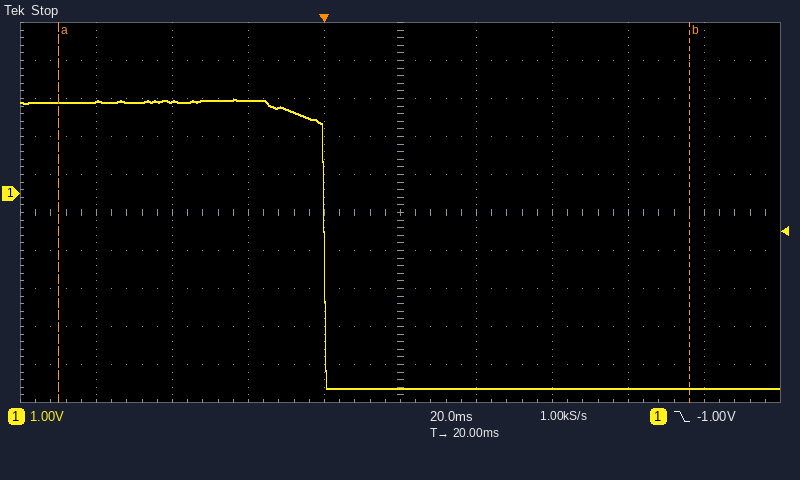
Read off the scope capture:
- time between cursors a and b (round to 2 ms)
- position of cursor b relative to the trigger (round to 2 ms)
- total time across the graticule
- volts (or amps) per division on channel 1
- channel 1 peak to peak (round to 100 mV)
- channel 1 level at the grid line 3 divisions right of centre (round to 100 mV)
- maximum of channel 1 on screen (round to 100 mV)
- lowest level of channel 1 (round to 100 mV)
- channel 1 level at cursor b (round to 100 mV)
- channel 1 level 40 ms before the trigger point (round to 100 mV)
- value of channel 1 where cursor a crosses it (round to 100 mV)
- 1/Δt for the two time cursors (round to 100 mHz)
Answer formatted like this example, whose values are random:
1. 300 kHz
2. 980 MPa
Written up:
1. 166 ms
2. +96 ms
3. 200 ms
4. 1 V
5. 7.6 V
6. -5.1 V
7. 2.5 V
8. -5.1 V
9. -5.1 V
10. 2.4 V
11. 2.4 V
12. 6.0 Hz
